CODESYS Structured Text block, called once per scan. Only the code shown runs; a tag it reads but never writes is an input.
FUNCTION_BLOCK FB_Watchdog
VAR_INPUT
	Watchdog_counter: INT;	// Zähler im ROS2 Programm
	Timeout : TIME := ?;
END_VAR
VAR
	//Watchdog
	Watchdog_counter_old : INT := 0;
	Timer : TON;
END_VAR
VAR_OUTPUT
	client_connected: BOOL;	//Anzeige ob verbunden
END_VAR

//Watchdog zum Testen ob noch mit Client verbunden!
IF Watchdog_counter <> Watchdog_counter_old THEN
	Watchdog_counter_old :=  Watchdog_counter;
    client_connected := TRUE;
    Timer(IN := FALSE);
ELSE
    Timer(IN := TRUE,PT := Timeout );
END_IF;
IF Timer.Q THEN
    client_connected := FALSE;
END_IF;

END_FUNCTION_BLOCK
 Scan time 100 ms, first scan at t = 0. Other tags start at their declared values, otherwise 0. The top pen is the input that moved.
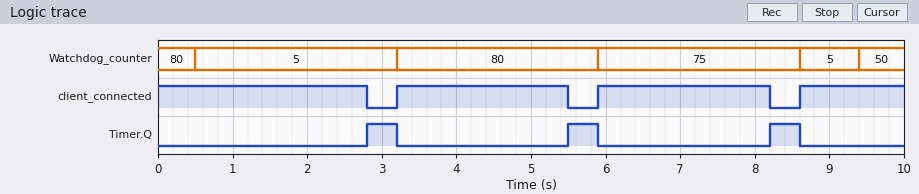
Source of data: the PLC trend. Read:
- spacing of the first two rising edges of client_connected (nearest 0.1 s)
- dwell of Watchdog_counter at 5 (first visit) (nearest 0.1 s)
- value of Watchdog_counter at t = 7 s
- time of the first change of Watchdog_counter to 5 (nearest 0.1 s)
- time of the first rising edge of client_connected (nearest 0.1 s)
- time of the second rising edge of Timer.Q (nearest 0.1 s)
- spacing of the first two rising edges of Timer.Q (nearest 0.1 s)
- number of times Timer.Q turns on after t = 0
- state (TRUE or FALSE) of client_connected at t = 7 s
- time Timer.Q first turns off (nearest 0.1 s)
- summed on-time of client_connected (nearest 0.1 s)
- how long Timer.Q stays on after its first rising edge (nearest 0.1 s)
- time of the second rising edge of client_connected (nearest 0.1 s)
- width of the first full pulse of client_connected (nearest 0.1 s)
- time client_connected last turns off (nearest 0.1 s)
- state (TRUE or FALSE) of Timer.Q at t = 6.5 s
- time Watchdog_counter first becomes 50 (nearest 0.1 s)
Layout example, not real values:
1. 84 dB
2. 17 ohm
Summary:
1. 2.7 s
2. 2.7 s
3. 75
4. 0.5 s
5. 3.2 s
6. 5.5 s
7. 2.7 s
8. 3
9. TRUE
10. 3.2 s
11. 8.8 s
12. 0.4 s
13. 5.9 s
14. 2.3 s
15. 8.2 s
16. FALSE
17. 9.4 s
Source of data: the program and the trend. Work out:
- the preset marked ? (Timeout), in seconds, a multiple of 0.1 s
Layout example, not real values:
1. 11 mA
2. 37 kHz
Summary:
1. 2.2 s
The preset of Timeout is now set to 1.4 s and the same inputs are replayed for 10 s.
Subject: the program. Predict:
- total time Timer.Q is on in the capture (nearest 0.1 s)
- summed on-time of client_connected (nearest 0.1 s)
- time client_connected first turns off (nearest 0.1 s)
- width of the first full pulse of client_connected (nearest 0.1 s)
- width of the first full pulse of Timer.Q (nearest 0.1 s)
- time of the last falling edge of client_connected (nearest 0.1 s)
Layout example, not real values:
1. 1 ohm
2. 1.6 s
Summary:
1. 3.6 s
2. 6.4 s
3. 2.0 s
4. 1.5 s
5. 1.2 s
6. 7.4 s
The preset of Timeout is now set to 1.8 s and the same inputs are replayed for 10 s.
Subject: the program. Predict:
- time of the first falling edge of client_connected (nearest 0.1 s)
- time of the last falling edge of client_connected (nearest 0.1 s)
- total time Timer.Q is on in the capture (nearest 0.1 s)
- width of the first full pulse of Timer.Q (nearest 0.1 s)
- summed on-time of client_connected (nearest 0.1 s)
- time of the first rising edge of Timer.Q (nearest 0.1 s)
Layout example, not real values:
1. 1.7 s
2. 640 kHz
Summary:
1. 2.4 s
2. 7.8 s
3. 2.4 s
4. 0.8 s
5. 7.6 s
6. 2.4 s
